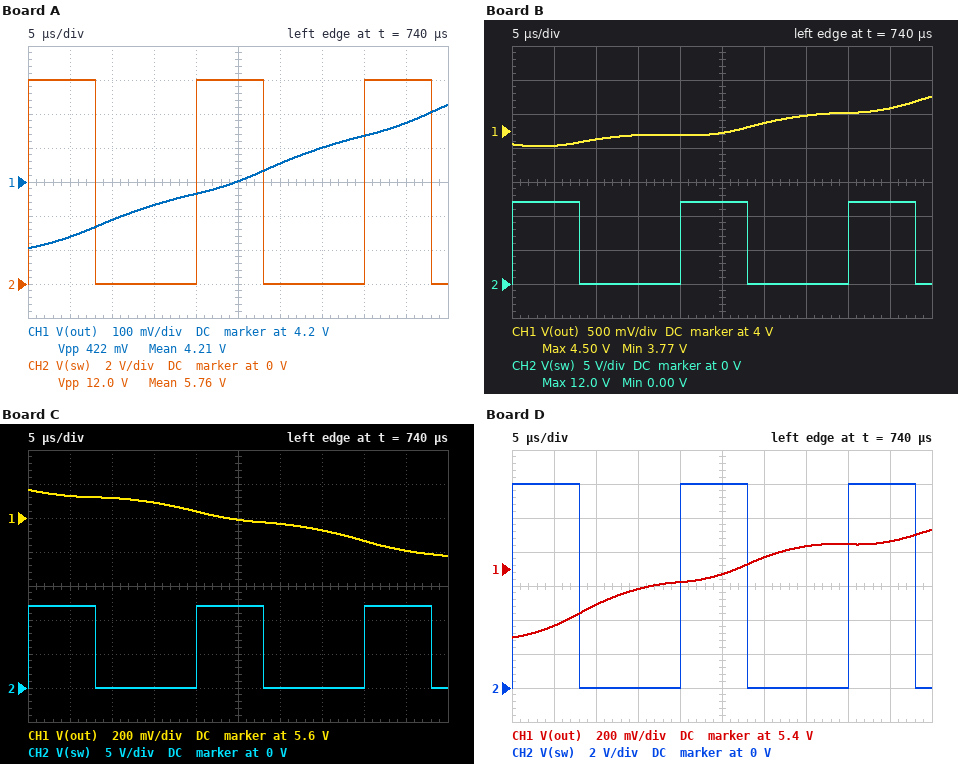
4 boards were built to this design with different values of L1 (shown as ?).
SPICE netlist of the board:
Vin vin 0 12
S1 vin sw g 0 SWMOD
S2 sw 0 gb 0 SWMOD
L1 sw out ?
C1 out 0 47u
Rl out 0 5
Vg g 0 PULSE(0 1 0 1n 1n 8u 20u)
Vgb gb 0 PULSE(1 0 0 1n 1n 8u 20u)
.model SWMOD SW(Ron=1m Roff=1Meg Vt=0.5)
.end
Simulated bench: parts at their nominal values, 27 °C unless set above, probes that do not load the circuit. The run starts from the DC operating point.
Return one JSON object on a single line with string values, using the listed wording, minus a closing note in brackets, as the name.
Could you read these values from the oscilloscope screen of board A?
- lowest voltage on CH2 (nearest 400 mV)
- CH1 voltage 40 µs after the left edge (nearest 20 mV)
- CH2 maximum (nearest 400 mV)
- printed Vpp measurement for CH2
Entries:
{"lowest voltage on CH2": "0 V", "CH1 voltage 40 µs after the left edge": "4.34 V", "CH2 maximum": "12.0 V", "printed Vpp measurement for CH2": "12.0 V"}
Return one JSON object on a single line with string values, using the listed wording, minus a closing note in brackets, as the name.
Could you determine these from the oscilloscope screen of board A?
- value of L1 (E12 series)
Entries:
{"value of L1": "220 µH"}
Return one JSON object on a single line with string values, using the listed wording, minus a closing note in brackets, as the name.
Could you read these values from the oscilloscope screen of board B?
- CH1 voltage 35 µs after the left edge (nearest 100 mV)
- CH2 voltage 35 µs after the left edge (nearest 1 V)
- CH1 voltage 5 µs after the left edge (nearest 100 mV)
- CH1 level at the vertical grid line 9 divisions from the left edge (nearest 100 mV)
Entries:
{"CH1 voltage 35 µs after the left edge": "4.2 V", "CH2 voltage 35 µs after the left edge": "0 V", "CH1 voltage 5 µs after the left edge": "3.8 V", "CH1 level at the vertical grid line 9 divisions from the left edge": "4.3 V"}
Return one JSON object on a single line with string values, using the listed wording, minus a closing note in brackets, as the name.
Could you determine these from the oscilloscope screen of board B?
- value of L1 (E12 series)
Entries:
{"value of L1": "33 µH"}
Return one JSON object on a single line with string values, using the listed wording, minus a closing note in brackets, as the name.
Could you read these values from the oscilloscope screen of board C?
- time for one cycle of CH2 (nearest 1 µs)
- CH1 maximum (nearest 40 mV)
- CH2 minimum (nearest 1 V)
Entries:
{"time for one cycle of CH2": "20 µs", "CH1 maximum": "5.76 V", "CH2 minimum": "0 V"}
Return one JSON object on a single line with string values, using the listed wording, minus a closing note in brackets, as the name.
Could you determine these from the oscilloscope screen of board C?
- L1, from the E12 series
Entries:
{"L1, from the E12 series": "120 µH"}
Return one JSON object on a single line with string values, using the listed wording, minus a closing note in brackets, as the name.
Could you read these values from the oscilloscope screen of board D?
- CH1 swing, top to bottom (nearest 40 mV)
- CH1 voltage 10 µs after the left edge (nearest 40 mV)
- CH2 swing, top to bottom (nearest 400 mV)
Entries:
{"CH1 swing, top to bottom": "640 mV", "CH1 voltage 10 µs after the left edge": "5.20 V", "CH2 swing, top to bottom": "12.0 V"}
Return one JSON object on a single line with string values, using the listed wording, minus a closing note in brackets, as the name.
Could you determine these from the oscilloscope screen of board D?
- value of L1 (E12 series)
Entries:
{"value of L1": "56 µH"}
